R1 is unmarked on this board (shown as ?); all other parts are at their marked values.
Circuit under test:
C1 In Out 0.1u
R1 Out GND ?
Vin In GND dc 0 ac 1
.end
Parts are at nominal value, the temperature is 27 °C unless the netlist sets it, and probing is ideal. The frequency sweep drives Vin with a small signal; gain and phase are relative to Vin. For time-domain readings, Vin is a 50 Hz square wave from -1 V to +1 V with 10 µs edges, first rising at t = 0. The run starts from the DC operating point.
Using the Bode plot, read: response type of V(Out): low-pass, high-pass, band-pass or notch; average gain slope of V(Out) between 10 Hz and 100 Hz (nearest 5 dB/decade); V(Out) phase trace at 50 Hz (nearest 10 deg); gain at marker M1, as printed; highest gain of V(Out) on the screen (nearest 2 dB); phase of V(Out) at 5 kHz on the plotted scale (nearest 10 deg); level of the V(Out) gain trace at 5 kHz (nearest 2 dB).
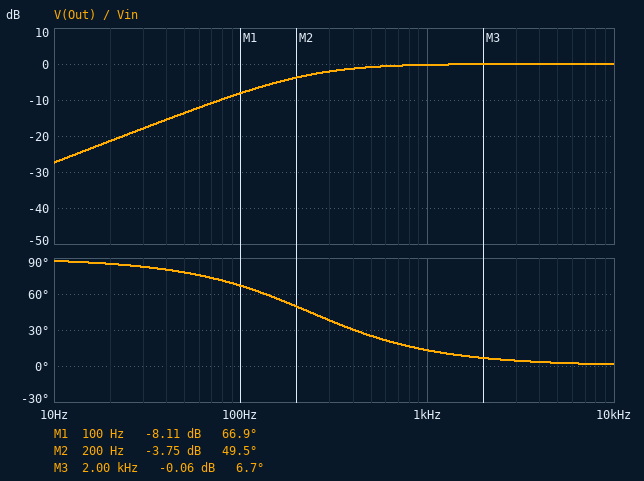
high-pass
20 dB/decade
80 deg
-8.11 dB
0 dB
0 deg
0 dB
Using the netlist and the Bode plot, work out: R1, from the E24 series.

6.8 kΩ
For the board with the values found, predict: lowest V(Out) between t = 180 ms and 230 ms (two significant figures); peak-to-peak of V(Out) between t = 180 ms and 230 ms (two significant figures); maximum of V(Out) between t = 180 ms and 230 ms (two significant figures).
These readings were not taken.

-2.0 V
4.0 V
2.0 V
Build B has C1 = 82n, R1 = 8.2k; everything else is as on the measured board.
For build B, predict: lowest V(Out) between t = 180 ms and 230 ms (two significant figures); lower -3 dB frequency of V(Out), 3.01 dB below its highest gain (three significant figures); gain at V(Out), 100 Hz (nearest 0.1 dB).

-2.0 V
237 Hz
-8.2 dB
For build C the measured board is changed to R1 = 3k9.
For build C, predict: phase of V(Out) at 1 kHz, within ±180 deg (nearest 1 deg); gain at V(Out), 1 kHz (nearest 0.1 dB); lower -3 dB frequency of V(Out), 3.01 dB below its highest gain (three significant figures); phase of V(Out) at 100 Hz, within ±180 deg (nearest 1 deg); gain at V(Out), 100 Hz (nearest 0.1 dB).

22 deg
-0.7 dB
408 Hz
76 deg
-12.5 dB
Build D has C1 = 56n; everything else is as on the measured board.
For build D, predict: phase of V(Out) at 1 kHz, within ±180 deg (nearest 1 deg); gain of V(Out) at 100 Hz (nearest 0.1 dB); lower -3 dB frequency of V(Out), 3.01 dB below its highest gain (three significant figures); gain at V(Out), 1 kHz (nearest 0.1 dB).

23 deg
-12.7 dB
418 Hz
-0.7 dB
